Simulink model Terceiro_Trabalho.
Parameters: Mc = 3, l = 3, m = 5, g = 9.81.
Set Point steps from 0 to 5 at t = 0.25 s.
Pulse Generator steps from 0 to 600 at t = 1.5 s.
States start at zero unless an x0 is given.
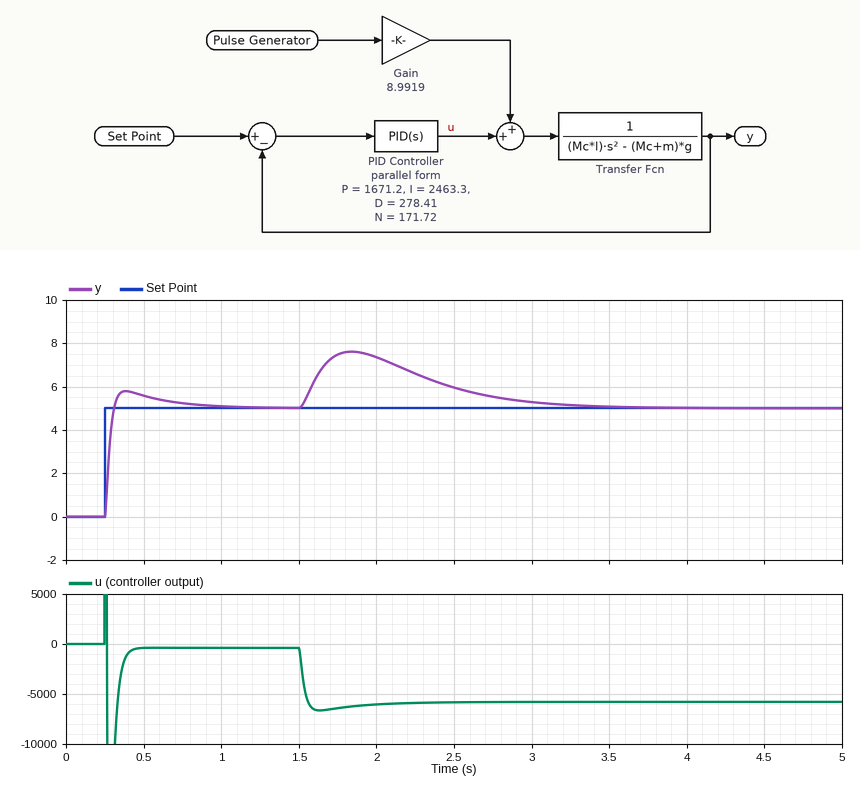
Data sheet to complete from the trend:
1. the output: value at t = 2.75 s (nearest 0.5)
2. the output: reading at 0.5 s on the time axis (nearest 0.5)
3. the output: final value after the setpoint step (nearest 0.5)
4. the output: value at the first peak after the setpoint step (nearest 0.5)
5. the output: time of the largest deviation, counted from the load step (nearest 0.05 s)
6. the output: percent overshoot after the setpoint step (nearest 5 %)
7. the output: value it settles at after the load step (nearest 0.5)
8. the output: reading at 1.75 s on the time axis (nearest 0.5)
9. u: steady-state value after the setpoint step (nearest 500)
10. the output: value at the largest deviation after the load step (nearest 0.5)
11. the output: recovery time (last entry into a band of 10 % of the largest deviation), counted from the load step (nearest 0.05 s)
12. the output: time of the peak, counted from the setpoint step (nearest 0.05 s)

5.5
5.5
5.0
6.0
0.35 s
15 %
5.0
7.5
-500
7.5
1.55 s
0.15 s
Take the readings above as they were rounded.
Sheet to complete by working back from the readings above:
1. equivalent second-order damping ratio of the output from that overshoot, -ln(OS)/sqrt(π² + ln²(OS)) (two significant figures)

0.52
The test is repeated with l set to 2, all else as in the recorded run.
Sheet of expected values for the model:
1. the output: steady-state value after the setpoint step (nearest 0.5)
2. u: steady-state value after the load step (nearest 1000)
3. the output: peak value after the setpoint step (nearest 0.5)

5.0
-6000
5.5
